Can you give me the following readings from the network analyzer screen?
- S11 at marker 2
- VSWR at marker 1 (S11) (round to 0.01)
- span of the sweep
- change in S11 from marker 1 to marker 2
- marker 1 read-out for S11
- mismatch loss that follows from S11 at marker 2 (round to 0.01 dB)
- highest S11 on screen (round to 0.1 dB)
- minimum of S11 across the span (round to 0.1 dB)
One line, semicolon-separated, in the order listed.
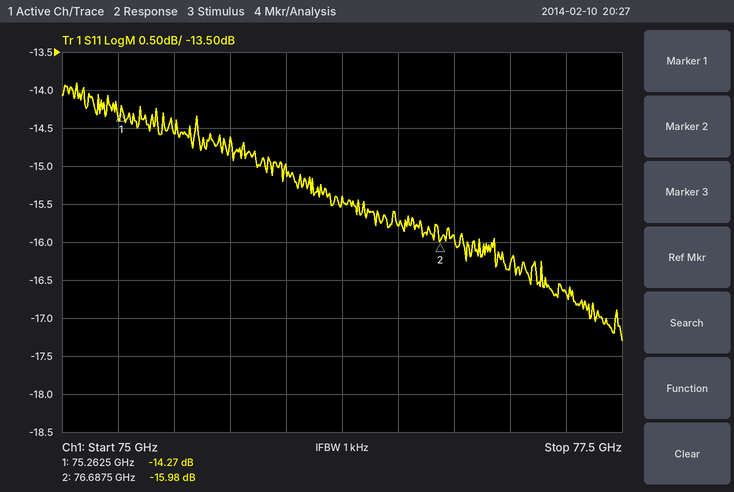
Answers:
-15.98 dB; 1.48; 2.5 GHz; -1.71 dB; -14.27 dB; 0.11 dB; -13.9 dB; -17.3 dB
